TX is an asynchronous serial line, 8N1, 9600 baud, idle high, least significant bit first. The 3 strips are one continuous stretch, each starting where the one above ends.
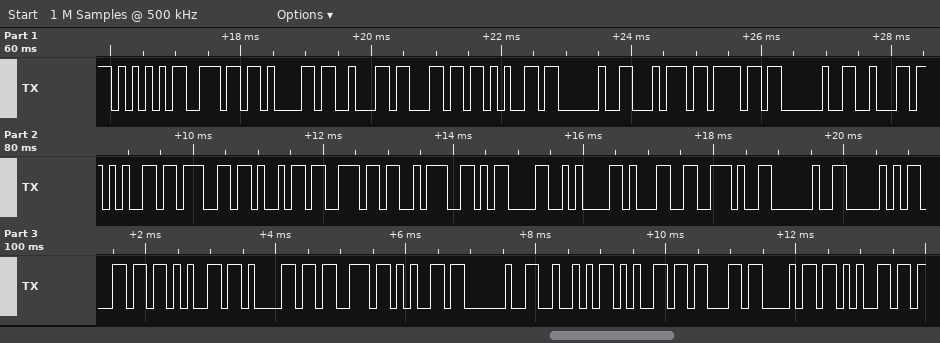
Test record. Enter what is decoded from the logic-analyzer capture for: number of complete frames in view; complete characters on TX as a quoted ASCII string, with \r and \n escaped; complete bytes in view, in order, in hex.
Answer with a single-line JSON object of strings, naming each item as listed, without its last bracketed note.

{"number of complete frames in view": "33", "complete characters on TX as a quoted ASCII string, with \\r and \\n escaped": "\"Unable to begin:\\r\\n1. Please Reche\"", "complete bytes in view, in order, in hex": "55 6E 61 62 6C 65 20 74 6F 20 62 65 67 69 6E 3A 0D 0A 31 2E 20 50 6C 65 61 73 65 20 52 65 63 68 65"}
